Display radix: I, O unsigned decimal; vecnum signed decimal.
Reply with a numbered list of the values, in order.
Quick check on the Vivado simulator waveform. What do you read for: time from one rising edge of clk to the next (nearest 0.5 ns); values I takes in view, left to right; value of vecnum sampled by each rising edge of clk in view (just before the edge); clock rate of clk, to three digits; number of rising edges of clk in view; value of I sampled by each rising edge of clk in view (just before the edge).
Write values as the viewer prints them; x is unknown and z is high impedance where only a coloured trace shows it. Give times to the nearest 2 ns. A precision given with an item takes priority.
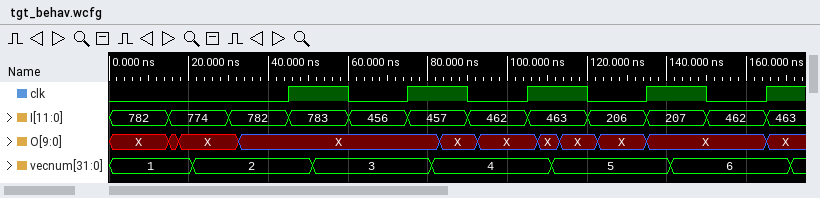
1. 30 ns
2. 782, 774, 782, 783, 456, 457, 462, 463, 206, 207, 462, 463
3. 2, 3, 4, 5, 6
4. 33.3 MHz
5. 5
6. 782, 456, 462, 206, 462
